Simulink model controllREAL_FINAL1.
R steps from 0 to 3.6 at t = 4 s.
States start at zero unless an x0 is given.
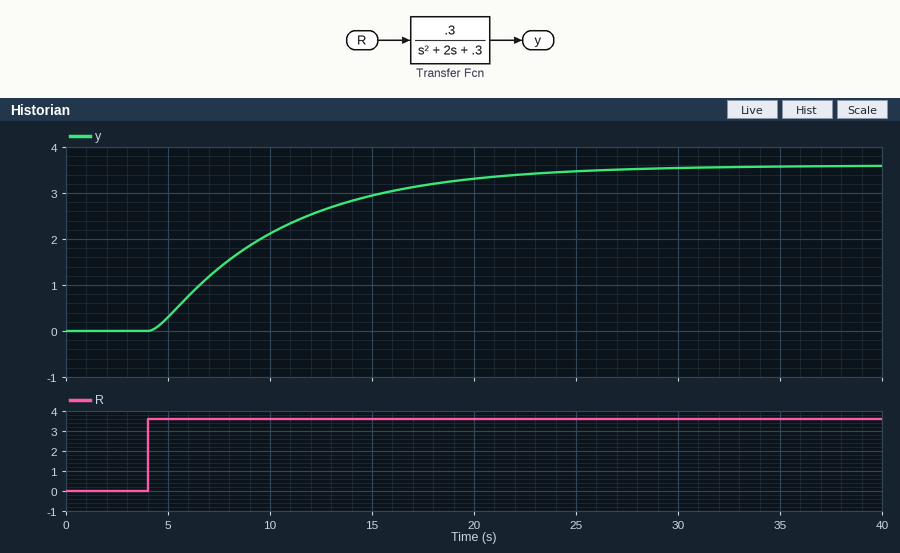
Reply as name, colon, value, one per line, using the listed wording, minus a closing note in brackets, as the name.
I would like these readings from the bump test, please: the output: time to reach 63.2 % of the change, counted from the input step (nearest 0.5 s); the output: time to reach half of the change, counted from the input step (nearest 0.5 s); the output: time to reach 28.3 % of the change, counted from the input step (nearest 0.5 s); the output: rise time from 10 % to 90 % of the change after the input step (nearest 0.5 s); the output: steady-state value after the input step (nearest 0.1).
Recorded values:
the output: time to reach 63.2 % of the change, counted from the input step: 6.5 s
the output: time to reach half of the change, counted from the input step: 5.0 s
the output: time to reach 28.3 % of the change, counted from the input step: 2.5 s
the output: rise time from 10 % to 90 % of the change after the input step: 13.5 s
the output: steady-state value after the input step: 3.6
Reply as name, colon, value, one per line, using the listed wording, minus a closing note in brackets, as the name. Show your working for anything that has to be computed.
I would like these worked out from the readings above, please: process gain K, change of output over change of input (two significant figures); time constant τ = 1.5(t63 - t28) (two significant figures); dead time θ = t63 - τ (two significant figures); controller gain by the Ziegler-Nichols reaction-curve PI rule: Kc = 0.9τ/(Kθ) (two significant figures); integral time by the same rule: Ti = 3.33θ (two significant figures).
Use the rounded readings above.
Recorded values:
process gain K, change of output over change of input: (3.6 - 0) / 3.6 = 1.0
time constant τ = 1.5(t63 - t28): 1.5 × (6.5 - 2.5) = 6.0 s
dead time θ = t63 - τ: 6.5 - 6 = 0.50 s
controller gain by the Ziegler-Nichols reaction-curve PI rule: Kc = 0.9τ/(Kθ): 0.9 × 6 / (1 × 0.5) = 11
integral time by the same rule: Ti = 3.33θ: 3.33 × 0.5 = 1.7 s
